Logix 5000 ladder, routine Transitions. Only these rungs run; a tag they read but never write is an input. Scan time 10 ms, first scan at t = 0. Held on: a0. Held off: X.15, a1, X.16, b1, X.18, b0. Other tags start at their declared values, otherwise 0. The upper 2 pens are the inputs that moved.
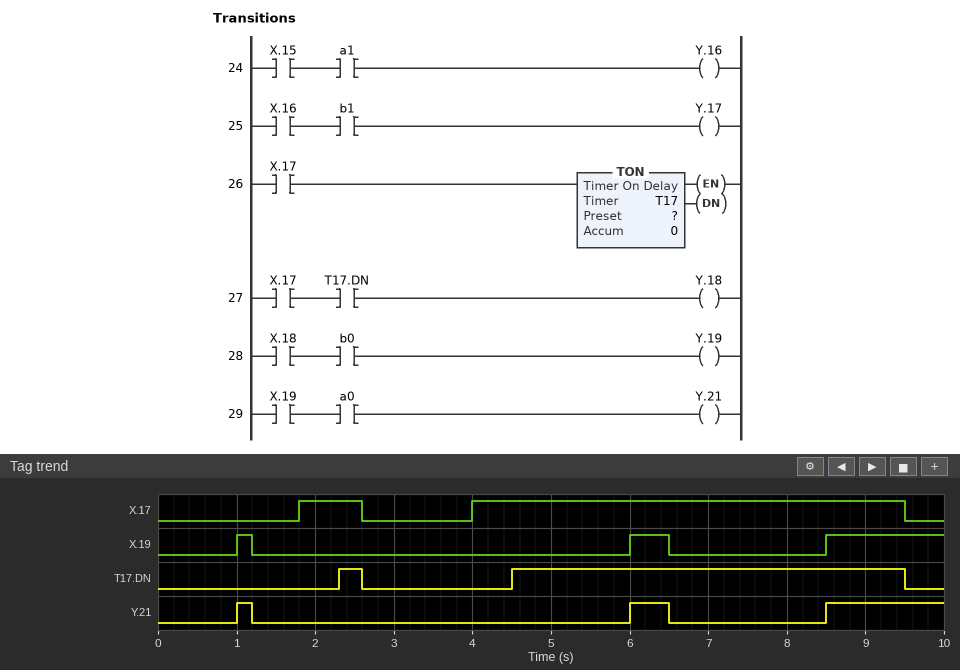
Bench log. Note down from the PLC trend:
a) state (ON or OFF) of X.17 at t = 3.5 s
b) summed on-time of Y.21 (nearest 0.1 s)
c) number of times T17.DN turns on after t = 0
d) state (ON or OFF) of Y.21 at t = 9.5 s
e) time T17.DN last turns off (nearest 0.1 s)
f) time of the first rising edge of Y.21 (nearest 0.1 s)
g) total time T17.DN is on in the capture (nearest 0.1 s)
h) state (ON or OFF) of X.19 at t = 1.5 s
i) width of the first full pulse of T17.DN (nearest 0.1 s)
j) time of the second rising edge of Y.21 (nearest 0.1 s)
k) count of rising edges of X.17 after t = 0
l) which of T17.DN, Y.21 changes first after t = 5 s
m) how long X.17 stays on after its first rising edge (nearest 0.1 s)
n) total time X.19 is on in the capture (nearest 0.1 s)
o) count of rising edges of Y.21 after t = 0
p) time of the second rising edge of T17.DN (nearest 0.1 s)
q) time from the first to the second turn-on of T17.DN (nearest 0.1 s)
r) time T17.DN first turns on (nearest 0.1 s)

OFF
2.2 s
2
ON
9.5 s
1.0 s
5.3 s
OFF
0.3 s
6.0 s
2
Y.21
0.8 s
2.2 s
3
4.5 s
2.2 s
2.3 s
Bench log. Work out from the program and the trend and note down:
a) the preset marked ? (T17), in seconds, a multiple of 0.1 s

0.5 s
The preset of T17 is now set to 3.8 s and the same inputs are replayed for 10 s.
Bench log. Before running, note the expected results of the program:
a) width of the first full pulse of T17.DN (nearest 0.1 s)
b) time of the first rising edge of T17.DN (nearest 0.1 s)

1.7 s
7.8 s
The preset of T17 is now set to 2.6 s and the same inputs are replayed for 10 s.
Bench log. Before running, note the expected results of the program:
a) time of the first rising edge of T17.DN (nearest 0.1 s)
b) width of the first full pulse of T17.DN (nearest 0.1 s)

6.6 s
2.9 s
